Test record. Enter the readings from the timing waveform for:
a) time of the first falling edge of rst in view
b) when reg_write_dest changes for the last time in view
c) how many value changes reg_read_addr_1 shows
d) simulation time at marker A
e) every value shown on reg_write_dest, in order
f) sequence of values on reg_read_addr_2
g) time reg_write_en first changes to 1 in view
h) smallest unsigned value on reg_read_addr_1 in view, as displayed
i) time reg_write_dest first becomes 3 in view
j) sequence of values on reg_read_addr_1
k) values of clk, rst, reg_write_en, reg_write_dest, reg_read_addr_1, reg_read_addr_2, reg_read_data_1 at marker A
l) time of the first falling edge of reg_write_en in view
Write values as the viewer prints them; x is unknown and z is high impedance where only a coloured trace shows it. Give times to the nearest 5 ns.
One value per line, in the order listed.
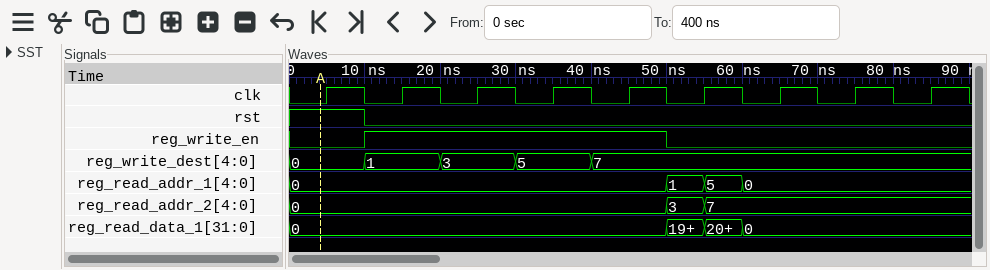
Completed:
10 ns
40 ns
3
5 ns
0, 1, 3, 5, 7
0, 3, 7
10 ns
0
20 ns
0, 1, 5, 0
clk=0, rst=1, reg_write_en=0, reg_write_dest=0, reg_read_addr_1=0, reg_read_addr_2=0, reg_read_data_1=0
50 ns
